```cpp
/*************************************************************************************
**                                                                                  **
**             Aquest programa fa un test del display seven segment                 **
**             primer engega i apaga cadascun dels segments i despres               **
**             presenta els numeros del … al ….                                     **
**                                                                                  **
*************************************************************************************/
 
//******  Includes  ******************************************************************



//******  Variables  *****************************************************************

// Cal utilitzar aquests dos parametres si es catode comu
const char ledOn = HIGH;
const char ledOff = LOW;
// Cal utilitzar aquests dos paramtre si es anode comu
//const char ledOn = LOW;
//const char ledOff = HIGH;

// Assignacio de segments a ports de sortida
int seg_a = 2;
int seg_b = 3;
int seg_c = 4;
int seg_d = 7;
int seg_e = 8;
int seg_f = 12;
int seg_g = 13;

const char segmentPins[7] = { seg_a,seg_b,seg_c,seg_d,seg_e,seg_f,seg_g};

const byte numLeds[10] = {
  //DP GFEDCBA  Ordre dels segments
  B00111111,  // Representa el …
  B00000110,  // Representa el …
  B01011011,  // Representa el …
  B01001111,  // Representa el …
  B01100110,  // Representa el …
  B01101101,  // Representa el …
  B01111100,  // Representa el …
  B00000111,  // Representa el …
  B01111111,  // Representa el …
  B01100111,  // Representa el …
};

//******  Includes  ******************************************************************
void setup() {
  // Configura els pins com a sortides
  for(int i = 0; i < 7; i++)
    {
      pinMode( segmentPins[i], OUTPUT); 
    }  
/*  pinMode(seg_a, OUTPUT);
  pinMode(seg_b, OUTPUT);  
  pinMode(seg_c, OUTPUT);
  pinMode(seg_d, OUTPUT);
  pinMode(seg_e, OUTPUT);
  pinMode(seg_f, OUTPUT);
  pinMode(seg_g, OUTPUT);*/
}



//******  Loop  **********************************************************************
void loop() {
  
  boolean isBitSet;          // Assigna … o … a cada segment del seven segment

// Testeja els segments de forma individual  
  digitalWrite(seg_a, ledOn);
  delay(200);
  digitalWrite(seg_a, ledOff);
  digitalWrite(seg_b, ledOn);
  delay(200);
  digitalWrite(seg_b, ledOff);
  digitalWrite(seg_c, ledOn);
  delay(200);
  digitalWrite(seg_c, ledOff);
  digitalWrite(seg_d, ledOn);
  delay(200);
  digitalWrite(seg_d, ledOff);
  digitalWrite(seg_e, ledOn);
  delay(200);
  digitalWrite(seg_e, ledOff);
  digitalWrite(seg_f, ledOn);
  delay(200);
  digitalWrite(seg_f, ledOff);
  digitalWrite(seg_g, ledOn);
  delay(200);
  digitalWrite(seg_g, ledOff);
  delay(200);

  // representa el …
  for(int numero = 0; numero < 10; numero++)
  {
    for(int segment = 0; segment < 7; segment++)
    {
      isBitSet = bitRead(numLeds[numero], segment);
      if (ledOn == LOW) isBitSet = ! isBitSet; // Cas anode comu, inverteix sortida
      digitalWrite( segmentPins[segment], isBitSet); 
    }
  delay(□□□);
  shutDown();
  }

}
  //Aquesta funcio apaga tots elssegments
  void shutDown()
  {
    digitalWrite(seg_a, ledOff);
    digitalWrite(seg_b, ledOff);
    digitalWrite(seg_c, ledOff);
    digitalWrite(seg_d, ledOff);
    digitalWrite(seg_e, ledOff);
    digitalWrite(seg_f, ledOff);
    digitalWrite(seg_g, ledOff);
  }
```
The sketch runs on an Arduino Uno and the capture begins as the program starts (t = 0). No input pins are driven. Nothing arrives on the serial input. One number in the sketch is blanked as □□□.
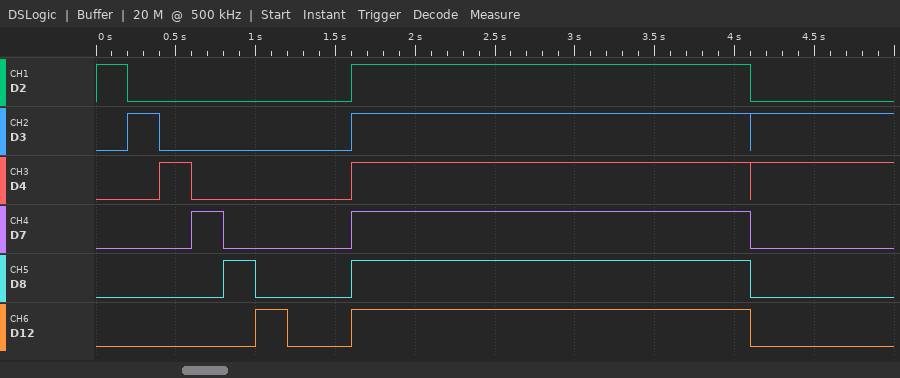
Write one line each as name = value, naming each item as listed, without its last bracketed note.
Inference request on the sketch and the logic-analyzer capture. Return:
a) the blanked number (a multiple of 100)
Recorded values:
the blanked number = 2500
